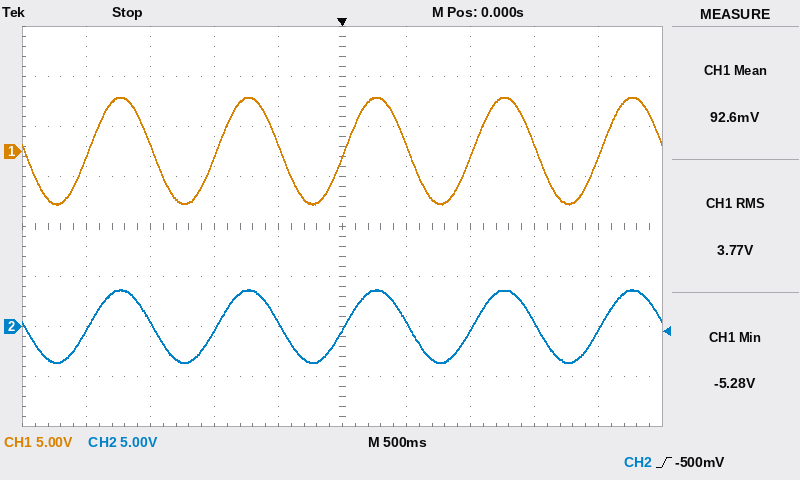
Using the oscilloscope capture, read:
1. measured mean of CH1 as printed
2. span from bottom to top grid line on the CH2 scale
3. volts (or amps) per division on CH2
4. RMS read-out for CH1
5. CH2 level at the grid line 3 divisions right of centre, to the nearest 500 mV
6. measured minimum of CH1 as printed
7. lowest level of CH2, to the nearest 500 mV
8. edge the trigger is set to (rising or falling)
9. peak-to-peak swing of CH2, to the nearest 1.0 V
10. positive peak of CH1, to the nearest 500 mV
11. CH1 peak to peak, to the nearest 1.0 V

92.6 mV
40 V
5 V
3.77 V
500 mV
-5.28 V
-3.5 V
rising
7.0 V
5.5 V
11.0 V
